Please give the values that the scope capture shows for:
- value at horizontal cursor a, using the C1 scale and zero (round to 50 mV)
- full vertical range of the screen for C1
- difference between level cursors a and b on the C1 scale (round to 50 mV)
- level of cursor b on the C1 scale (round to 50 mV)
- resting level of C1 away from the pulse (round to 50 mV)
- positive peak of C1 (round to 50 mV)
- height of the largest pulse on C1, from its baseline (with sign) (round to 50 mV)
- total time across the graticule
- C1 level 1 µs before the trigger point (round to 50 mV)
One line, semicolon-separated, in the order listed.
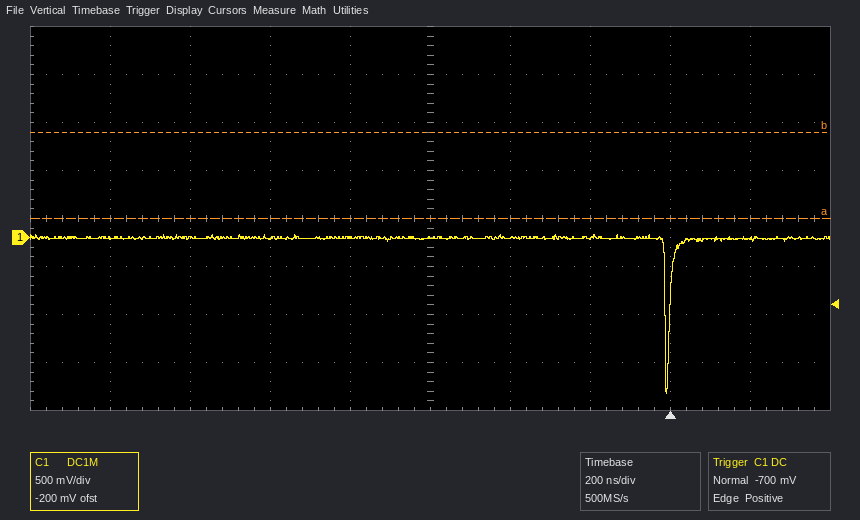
200 mV; 4 V; 900 mV; 1.10 V; 0 mV; 50 mV; -1.60 V; 2 µs; 0 mV
